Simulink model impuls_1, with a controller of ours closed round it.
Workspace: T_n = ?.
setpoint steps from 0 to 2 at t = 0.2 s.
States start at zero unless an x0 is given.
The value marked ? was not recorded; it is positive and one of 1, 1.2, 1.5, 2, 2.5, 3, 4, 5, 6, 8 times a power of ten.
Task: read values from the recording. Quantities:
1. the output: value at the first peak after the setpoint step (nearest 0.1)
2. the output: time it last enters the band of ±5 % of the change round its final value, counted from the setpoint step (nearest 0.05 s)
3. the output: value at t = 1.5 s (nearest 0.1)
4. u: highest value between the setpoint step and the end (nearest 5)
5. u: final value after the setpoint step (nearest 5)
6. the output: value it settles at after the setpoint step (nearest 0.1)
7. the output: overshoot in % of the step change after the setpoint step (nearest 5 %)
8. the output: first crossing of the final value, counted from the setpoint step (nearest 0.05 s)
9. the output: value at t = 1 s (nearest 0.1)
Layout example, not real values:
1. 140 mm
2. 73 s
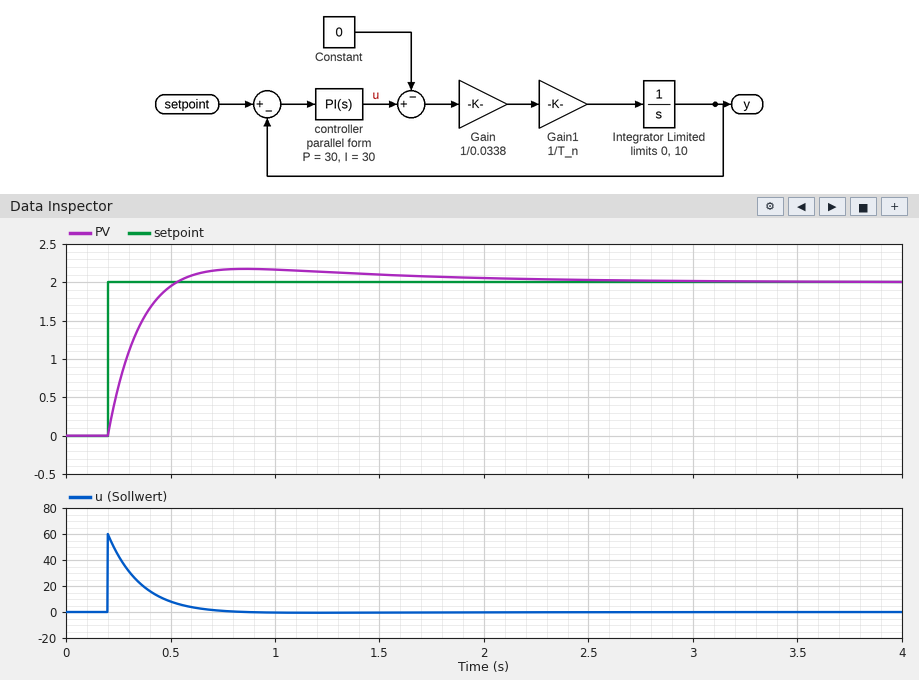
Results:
1. 2.2
2. 1.30 s
3. 2.1
4. 60
5. 0
6. 2.0
7. 10 %
8. 0.35 s
9. 2.2
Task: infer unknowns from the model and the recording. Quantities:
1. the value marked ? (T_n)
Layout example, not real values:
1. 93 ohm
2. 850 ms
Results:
1. 120
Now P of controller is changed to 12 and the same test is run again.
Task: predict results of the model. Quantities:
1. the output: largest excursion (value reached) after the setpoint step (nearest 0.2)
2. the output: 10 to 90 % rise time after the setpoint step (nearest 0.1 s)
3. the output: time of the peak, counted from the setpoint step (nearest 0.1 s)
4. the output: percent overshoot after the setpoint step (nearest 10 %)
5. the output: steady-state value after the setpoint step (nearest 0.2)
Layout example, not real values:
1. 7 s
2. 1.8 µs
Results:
1. 2.6
2. 0.3 s
3. 0.9 s
4. 30 %
5. 2.0
